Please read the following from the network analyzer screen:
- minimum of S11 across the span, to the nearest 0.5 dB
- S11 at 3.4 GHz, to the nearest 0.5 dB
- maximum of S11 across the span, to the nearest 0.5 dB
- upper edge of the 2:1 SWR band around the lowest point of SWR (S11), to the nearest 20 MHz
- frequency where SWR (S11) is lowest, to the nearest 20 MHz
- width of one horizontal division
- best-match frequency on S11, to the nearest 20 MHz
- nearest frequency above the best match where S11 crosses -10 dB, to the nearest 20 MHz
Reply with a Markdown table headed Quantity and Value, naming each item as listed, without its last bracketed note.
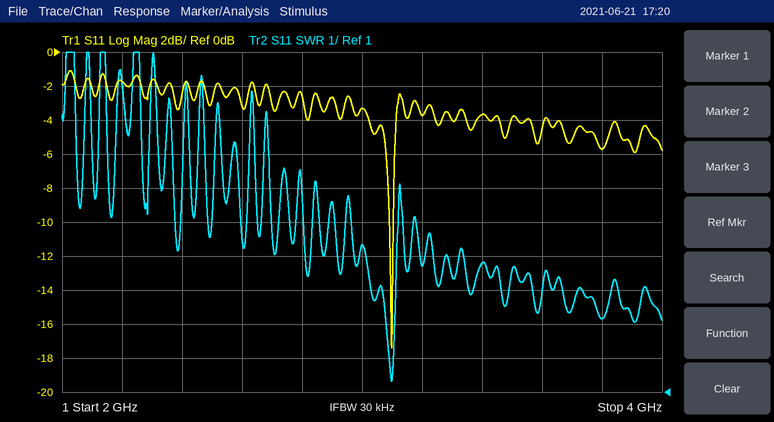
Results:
| Quantity | Value |
|---|---|
| minimum of S11 across the span, to the nearest 0.5 dB | -17.5 dB |
| S11 at 3.4 GHz, to the nearest 0.5 dB | -3.5 dB |
| maximum of S11 across the span, to the nearest 0.5 dB | -1.0 dB |
| upper edge of the 2:1 SWR band around the lowest point of SWR (S11), to the nearest 20 MHz | 3.10 GHz |
| frequency where SWR (S11) is lowest, to the nearest 20 MHz | 3.10 GHz |
| width of one horizontal division | 200 MHz |
| best-match frequency on S11, to the nearest 20 MHz | 3.10 GHz |
| nearest frequency above the best match where S11 crosses -10 dB, to the nearest 20 MHz | 3.10 GHz |
